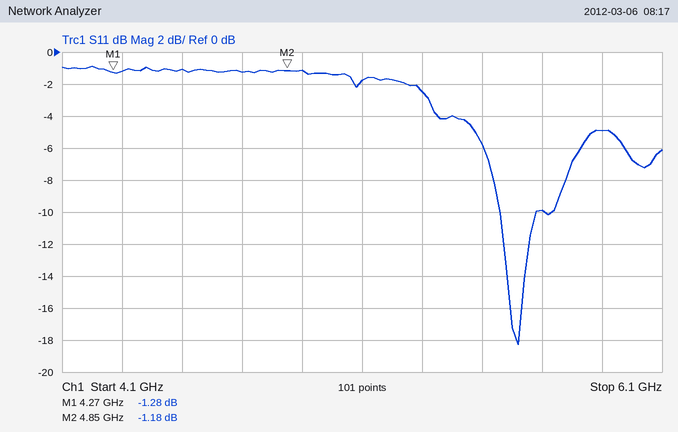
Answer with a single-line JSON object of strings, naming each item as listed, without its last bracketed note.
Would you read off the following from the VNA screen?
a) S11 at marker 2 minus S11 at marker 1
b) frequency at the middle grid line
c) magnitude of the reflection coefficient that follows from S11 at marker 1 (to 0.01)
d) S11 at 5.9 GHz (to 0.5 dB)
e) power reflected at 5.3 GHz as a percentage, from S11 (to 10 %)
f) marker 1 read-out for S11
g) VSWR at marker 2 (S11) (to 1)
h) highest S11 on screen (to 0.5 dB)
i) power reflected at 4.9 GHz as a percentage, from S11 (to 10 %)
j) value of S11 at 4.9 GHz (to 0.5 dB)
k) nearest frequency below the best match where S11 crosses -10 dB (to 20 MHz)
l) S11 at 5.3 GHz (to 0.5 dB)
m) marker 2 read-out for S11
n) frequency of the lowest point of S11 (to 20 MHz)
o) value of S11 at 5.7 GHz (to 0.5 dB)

{"S11 at marker 2 minus S11 at marker 1": "0.10 dB", "frequency at the middle grid line": "5.1 GHz", "magnitude of the reflection coefficient that follows from S11 at marker 1": "0.86", "S11 at 5.9 GHz": "-5.0 dB", "power reflected at 5.3 GHz as a percentage, from S11": "60 %", "marker 1 read-out for S11": "-1.28 dB", "VSWR at marker 2 (S11)": "15", "highest S11 on screen": "-1.0 dB", "power reflected at 4.9 GHz as a percentage, from S11": "80 %", "value of S11 at 4.9 GHz": "-1.0 dB", "nearest frequency below the best match where S11 crosses -10 dB": "5.56 GHz", "S11 at 5.3 GHz": "-2.5 dB", "marker 2 read-out for S11": "-1.18 dB", "frequency of the lowest point of S11": "5.62 GHz", "value of S11 at 5.7 GHz": "-10.0 dB"}
